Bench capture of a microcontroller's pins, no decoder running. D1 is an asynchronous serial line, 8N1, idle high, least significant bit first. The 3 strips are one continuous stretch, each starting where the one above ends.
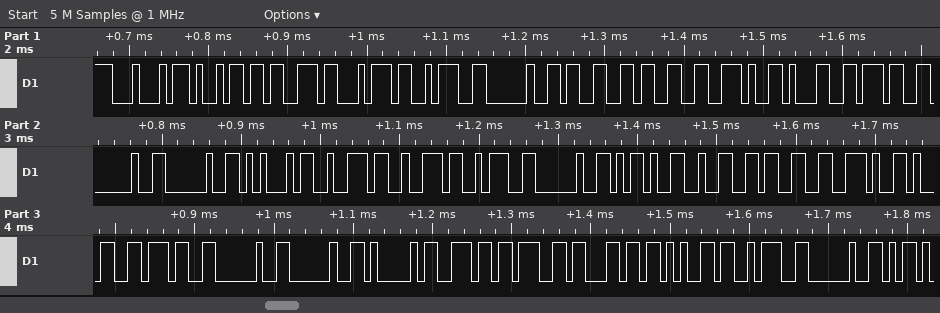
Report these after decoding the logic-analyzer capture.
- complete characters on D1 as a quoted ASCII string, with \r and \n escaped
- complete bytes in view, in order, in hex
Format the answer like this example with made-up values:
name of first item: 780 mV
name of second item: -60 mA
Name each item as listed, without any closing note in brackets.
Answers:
complete characters on D1 as a quoted ASCII string, with \r and \n escaped: "Dist: 33.17  Err: -23.17  Angle: "
complete bytes in view, in order, in hex: 44 69 73 74 3A 20 33 33 2E 31 37 20 20 45 72 72 3A 20 2D 32 33 2E 31 37 20 20 41 6E 67 6C 65 3A 20
